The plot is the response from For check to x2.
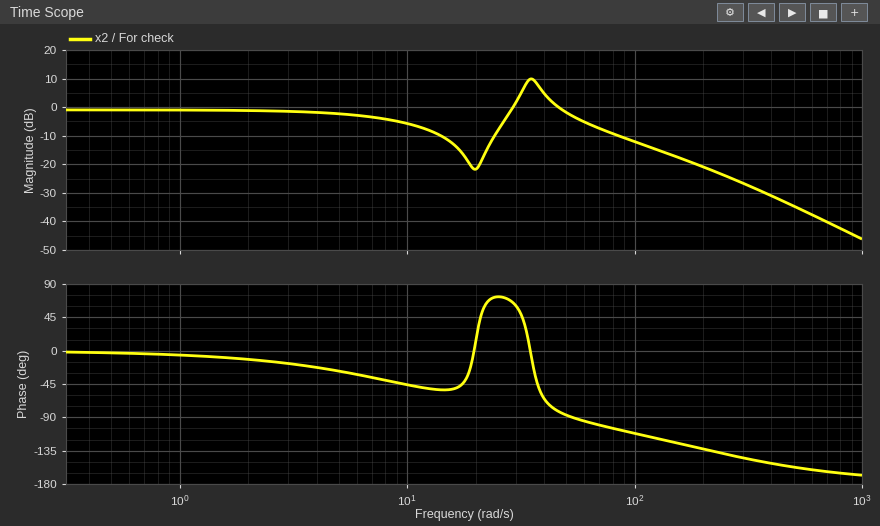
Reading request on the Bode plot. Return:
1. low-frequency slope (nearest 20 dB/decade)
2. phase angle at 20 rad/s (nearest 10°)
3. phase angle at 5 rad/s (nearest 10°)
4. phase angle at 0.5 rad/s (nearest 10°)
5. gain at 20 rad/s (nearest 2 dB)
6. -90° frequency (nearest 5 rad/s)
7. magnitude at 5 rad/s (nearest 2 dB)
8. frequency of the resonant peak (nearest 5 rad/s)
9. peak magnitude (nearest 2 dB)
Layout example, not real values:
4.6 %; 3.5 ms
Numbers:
0 dB/decade; 10°; -30°; 0°; -22 dB; 55 rad/s; -2 dB; 35 rad/s; 10 dB
